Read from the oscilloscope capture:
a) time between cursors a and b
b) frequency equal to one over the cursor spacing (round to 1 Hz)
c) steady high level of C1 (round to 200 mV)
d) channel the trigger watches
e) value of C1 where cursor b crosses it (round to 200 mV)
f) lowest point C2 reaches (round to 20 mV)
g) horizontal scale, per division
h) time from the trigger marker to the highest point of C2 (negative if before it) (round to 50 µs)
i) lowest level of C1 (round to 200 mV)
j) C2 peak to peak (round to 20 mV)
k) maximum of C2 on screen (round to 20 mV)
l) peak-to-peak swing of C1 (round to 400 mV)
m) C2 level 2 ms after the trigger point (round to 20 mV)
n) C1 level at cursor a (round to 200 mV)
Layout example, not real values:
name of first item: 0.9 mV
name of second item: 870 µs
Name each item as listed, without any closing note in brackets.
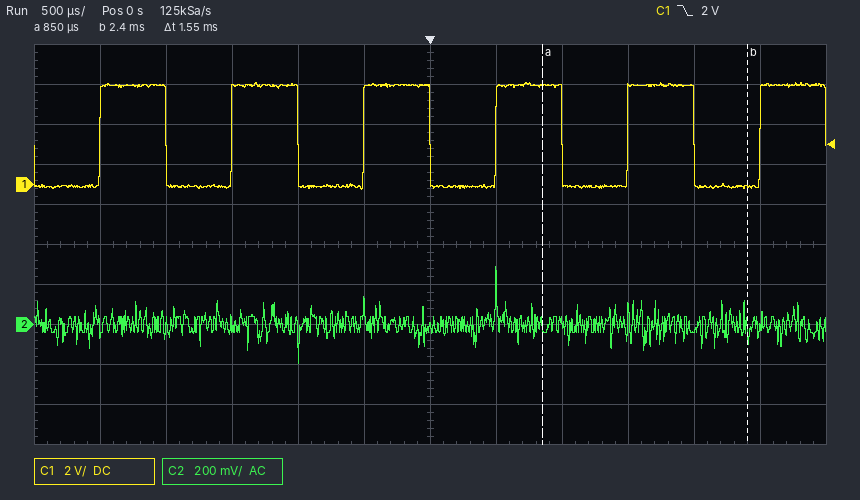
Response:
time between cursors a and b: 1.55 ms
frequency equal to one over the cursor spacing: 645 Hz
steady high level of C1: 5.0 V
channel the trigger watches: C1
value of C1 where cursor b crosses it: -200 mV
lowest point C2 reaches: -200 mV
horizontal scale, per division: 500 µs
time from the trigger marker to the highest point of C2 (negative if before it): +500 µs
lowest level of C1: -200 mV
C2 peak to peak: 480 mV
maximum of C2 on screen: 280 mV
peak-to-peak swing of C1: 5.2 V
C2 level 2 ms after the trigger point: -20 mV
C1 level at cursor a: 5.0 V
